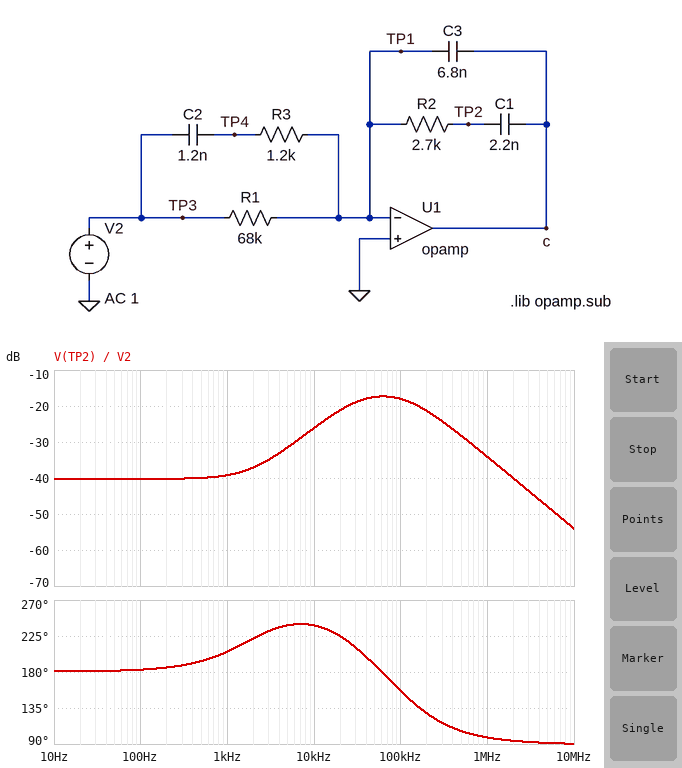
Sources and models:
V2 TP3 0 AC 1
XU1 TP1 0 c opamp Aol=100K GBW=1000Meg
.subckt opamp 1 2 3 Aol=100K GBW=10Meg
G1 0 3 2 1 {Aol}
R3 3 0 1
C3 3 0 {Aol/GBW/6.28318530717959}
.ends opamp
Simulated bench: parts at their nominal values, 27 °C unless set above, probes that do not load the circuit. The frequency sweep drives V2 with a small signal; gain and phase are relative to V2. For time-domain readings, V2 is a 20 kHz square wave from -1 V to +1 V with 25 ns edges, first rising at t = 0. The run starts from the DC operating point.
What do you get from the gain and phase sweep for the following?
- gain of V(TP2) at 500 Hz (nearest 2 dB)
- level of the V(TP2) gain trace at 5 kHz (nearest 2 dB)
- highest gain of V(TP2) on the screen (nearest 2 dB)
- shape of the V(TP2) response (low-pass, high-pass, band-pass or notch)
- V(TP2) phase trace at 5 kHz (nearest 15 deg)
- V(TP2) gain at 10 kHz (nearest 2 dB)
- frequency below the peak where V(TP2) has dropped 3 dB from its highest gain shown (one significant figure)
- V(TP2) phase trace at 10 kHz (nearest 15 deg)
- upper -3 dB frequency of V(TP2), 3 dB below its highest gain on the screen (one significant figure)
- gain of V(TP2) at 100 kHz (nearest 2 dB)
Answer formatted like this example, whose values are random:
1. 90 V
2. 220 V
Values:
1. -40 dB
2. -32 dB
3. -18 dB
4. band-pass
5. 240 deg
6. -26 dB
7. 20 kHz
8. 240 deg
9. 200 kHz
10. -18 dB
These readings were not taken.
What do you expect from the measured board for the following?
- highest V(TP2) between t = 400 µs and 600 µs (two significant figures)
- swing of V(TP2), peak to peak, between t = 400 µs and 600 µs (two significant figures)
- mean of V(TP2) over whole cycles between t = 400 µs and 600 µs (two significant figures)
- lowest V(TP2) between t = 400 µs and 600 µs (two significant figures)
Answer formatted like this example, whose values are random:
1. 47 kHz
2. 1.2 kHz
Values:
1. -810 mV
2. 410 mV
3. -1.0 V
4. -1.2 V
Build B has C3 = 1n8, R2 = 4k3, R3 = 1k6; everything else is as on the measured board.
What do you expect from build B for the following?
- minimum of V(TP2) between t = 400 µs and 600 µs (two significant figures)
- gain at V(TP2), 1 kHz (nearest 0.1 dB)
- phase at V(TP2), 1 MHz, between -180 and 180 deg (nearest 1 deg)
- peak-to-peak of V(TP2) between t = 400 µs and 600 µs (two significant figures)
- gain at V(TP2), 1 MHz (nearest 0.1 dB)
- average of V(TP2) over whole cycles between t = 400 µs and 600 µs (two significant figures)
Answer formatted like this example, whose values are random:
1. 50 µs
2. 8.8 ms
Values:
1. -1.7 V
2. -28.1 dB
3. 97 deg
4. 1.4 V
5. -25.0 dB
6. -1.0 V
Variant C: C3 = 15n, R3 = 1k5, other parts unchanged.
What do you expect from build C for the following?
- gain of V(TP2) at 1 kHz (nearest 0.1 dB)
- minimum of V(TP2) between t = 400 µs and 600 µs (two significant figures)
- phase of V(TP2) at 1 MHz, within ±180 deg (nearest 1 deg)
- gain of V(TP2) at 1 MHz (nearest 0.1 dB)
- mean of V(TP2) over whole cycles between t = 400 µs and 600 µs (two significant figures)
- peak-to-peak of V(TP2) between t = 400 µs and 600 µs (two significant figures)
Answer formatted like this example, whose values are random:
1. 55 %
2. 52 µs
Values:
1. -44.8 dB
2. -1.1 V
3. 97 deg
4. -42.9 dB
5. -1.0 V
6. 180 mV
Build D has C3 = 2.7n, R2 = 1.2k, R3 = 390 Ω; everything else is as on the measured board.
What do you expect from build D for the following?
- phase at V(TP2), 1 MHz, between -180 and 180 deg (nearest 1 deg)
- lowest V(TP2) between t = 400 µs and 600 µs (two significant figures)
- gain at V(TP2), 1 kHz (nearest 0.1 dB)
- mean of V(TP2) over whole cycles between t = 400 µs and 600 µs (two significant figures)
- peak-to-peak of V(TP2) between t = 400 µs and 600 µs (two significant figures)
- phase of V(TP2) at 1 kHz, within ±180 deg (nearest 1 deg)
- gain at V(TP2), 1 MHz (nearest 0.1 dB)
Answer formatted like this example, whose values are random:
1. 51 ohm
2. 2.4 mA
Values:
1. 115 deg
2. -1.5 V
3. -41.0 dB
4. -1.0 V
5. 1.0 V
6. -153 deg
7. -16.9 dB
